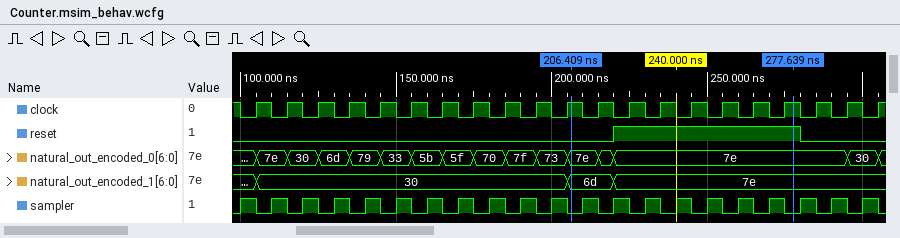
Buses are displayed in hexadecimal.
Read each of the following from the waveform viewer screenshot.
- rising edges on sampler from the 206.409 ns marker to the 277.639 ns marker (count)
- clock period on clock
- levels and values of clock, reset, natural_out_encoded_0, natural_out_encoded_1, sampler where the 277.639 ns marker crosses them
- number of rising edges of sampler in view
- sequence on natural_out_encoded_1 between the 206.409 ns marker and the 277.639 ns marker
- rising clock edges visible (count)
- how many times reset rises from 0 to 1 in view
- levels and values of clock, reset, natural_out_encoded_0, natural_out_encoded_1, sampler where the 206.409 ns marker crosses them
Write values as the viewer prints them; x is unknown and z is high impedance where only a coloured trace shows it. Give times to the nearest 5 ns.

7
10 ns
clock=1, reset=1, natural_out_encoded_0=7e, natural_out_encoded_1=7e, sampler=0
21
6d, 7e
21
1
clock=1, reset=0, natural_out_encoded_0=7e, natural_out_encoded_1=6d, sampler=0
